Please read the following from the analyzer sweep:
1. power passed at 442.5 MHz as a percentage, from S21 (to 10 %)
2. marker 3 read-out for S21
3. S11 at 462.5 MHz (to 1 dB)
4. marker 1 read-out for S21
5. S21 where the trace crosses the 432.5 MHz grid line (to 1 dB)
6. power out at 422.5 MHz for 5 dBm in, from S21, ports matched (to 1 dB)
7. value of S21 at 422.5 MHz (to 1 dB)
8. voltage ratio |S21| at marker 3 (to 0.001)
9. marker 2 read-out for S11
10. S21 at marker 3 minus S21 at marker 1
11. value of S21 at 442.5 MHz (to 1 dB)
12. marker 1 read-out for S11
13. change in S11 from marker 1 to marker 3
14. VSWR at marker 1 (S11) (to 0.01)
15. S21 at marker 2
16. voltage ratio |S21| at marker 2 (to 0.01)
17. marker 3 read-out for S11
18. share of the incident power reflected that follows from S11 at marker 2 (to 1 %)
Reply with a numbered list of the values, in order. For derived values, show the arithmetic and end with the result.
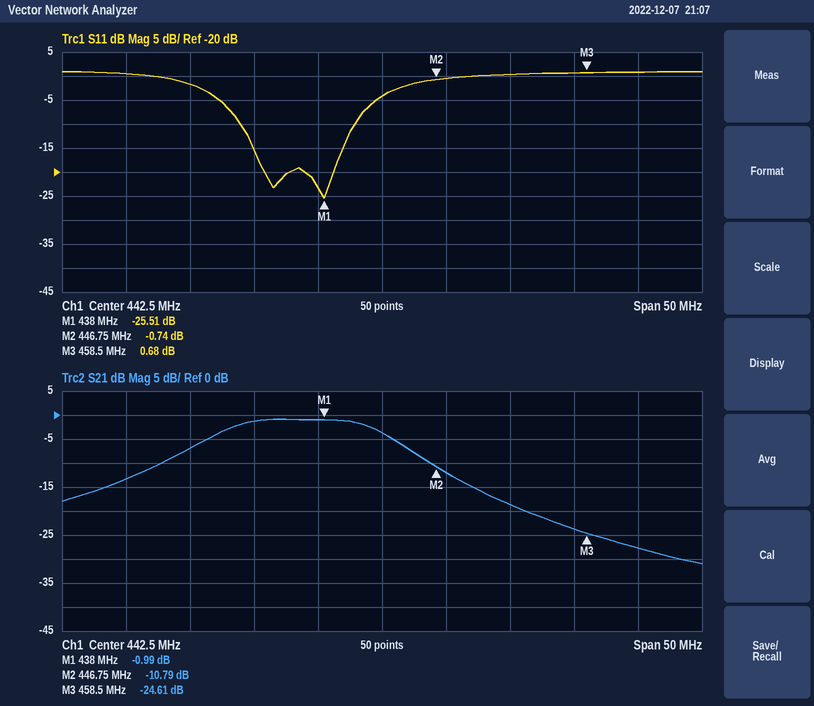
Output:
1. 10^(-4/10) ≈ 40 %
2. -24.61 dB
3. 1 dB
4. -0.99 dB
5. -1 dB
6. 5 dBm + (-13 dB) = -8 dBm
7. -13 dB
8. 10^(-24.61/20) ≈ 0.059
9. -0.74 dB
10. -24.61 − (-0.99) = -23.62 dB
11. -4 dB
12. -25.51 dB
13. 0.68 − (-25.51) = 26.19 dB
14. (1 + 0.0530)/(1 − 0.0530) ≈ 1.11
15. -10.79 dB
16. 10^(-10.79/20) ≈ 0.29
17. 0.68 dB
18. 10^(-0.74/10) ≈ 84 %
